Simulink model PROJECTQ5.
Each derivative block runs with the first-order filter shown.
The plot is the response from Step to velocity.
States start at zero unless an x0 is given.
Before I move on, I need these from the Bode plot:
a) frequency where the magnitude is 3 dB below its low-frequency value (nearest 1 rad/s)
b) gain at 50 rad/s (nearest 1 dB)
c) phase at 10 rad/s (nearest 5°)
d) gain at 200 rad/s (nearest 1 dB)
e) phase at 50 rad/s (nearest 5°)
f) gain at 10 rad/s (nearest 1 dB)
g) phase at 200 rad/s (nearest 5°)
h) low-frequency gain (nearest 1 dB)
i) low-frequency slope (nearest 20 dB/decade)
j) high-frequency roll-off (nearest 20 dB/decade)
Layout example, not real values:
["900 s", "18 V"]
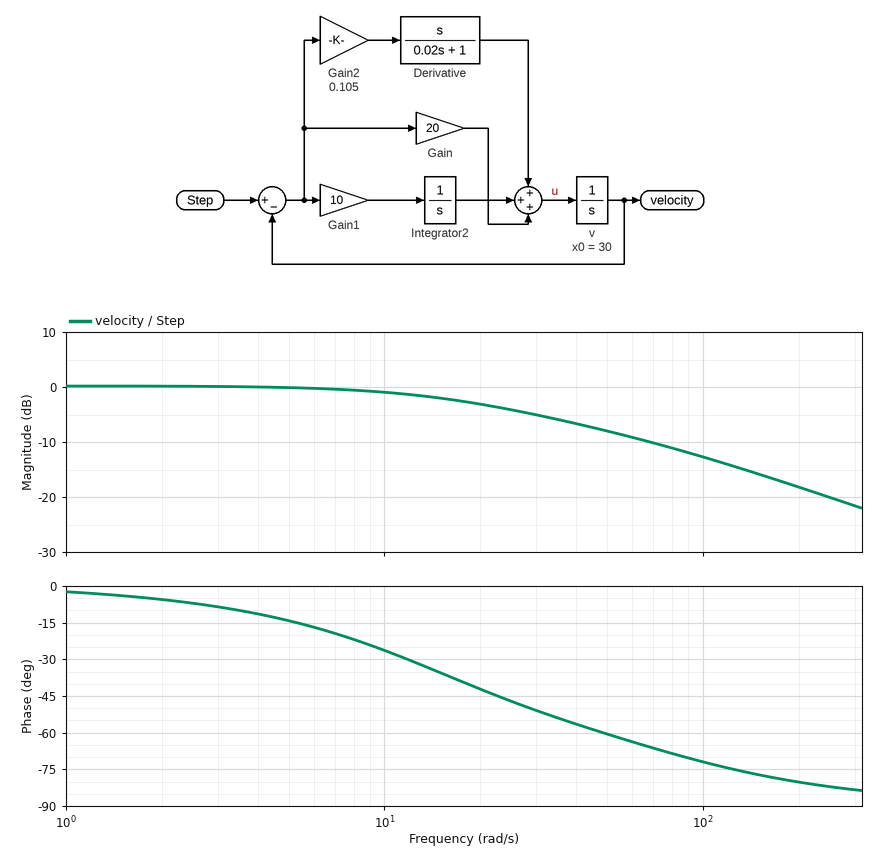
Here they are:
["19 rad/s", "-8 dB", "-25°", "-18 dB", "-60°", "-1 dB", "-80°", "0 dB", "0 dB/decade", "-20 dB/decade"]
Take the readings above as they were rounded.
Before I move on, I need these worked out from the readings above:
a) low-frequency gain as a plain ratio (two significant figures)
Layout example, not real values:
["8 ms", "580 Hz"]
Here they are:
["1.0"]
